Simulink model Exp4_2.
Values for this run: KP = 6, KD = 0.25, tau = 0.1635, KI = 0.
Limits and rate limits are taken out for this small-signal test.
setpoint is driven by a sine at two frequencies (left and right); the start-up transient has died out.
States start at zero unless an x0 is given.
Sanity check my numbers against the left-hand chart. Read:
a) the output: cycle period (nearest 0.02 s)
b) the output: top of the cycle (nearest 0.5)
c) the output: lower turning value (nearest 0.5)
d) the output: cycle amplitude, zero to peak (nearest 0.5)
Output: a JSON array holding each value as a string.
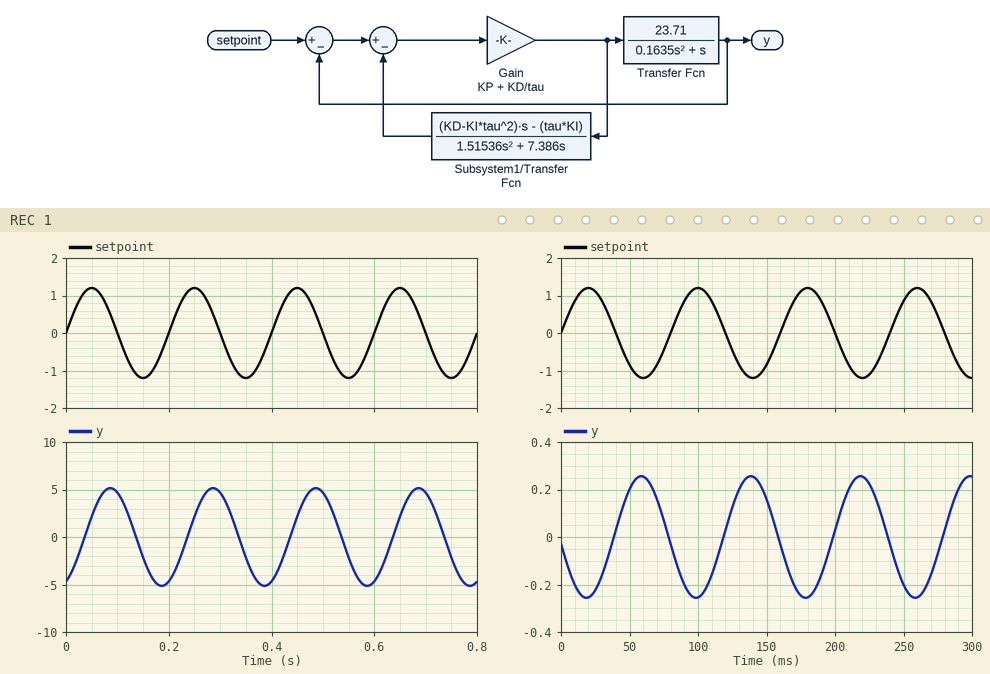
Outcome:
["0.20 s", "5.0", "-5.0", "5.0"]
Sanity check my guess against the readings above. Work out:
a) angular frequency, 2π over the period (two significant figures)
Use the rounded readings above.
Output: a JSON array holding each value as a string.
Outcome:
["31 rad/s"]
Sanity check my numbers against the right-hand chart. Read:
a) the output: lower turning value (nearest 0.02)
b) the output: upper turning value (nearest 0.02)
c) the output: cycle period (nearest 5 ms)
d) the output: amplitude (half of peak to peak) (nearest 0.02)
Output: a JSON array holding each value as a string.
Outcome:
["-0.26", "0.26", "80 ms", "0.26"]
